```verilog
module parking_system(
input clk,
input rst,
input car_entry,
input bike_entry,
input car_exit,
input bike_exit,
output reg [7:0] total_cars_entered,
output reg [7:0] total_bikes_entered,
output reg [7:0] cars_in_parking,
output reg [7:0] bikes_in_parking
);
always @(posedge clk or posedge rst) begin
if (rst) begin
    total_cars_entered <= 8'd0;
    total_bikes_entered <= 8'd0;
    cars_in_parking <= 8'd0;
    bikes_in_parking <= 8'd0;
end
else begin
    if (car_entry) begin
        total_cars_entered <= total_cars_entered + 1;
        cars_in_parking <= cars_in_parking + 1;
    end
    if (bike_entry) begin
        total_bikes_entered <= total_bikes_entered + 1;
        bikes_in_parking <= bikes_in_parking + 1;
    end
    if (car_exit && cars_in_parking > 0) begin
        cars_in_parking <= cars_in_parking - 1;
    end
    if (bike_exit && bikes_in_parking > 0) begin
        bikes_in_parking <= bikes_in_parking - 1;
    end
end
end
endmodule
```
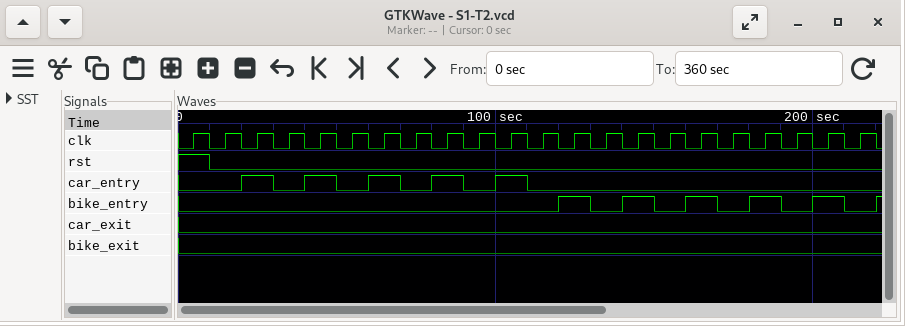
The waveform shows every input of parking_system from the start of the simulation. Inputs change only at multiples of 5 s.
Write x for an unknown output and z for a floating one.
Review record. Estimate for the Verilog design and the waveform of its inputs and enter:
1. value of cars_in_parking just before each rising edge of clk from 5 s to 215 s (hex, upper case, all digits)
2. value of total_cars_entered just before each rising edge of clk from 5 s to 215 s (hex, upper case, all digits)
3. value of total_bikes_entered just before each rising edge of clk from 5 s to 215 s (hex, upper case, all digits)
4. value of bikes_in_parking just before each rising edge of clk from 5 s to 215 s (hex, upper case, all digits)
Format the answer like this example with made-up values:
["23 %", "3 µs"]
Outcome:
["00, 00, 00, 01, 01, 02, 02, 03, 03, 04, 04, 05, 05, 05, 05, 05, 05, 05, 05, 05, 05, 05", "00, 00, 00, 01, 01, 02, 02, 03, 03, 04, 04, 05, 05, 05, 05, 05, 05, 05, 05, 05, 05, 05", "00, 00, 00, 00, 00, 00, 00, 00, 00, 00, 00, 00, 00, 01, 01, 02, 02, 03, 03, 04, 04, 05", "00, 00, 00, 00, 00, 00, 00, 00, 00, 00, 00, 00, 00, 01, 01, 02, 02, 03, 03, 04, 04, 05"]
